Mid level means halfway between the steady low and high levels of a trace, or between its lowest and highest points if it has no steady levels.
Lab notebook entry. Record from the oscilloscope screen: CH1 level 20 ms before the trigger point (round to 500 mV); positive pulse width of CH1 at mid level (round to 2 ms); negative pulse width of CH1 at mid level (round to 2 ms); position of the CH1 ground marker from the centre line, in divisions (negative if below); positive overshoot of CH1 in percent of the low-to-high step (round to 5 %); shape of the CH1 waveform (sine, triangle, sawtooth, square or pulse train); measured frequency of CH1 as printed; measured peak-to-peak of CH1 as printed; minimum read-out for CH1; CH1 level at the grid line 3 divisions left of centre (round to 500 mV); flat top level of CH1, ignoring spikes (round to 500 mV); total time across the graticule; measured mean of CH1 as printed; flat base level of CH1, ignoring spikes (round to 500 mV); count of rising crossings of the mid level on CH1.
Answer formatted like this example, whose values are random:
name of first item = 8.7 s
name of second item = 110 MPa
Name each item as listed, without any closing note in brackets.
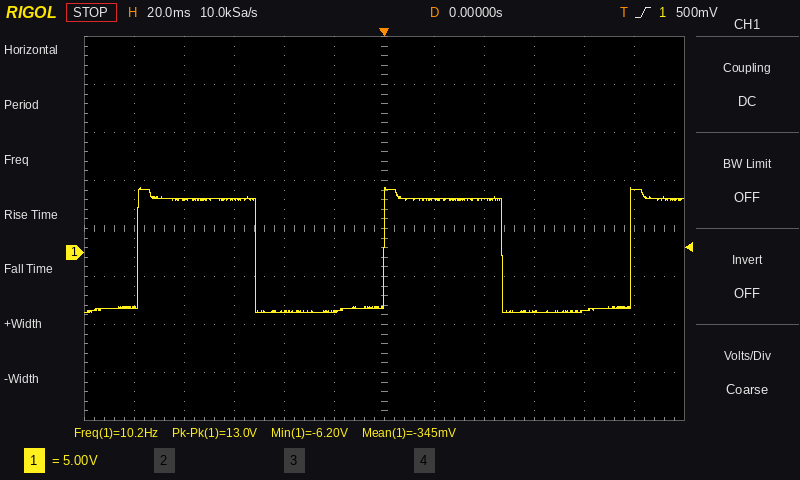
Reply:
CH1 level 20 ms before the trigger point = -6.0 V
positive pulse width of CH1 at mid level = 48 ms
negative pulse width of CH1 at mid level = 52 ms
position of the CH1 ground marker from the centre line, in divisions = -0.5 div
positive overshoot of CH1 in percent of the low-to-high step = 10 %
shape of the CH1 waveform = square
measured frequency of CH1 as printed = 10.2 Hz
measured peak-to-peak of CH1 as printed = 13.0 V
minimum read-out for CH1 = -6.20 V
CH1 level at the grid line 3 divisions left of centre = 5.5 V
flat top level of CH1, ignoring spikes = 5.5 V
total time across the graticule = 240 ms
measured mean of CH1 as printed = -345 mV
flat base level of CH1, ignoring spikes = -6.0 V
count of rising crossings of the mid level on CH1 = 3
